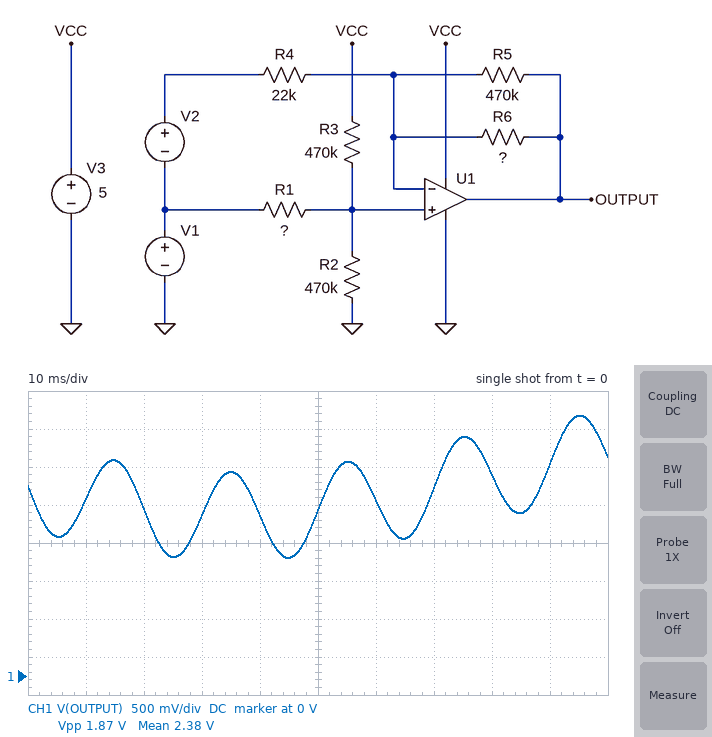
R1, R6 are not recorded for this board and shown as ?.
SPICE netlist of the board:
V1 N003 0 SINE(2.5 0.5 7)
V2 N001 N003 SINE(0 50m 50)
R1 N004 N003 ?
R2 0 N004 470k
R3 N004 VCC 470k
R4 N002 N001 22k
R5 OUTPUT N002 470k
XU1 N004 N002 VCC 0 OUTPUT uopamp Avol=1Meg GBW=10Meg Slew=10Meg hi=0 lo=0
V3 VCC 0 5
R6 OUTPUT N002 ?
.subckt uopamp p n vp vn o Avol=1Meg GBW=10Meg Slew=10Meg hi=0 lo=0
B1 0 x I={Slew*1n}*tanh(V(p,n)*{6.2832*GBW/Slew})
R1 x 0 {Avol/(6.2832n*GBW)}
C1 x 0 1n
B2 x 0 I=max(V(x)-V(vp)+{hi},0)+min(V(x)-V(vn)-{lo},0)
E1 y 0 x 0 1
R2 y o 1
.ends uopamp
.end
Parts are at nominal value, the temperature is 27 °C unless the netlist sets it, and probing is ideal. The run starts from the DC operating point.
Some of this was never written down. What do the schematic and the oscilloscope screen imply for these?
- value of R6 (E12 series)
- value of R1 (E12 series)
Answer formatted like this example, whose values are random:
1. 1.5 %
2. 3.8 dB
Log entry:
1. 560 kΩ
2. 39 kΩ
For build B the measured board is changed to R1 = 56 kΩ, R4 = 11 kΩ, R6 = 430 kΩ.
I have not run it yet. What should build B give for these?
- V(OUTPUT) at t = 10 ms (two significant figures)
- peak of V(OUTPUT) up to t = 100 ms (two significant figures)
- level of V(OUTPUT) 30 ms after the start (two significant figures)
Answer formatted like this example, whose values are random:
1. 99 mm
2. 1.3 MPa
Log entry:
1. 1.8 V
2. 4.9 V
3. 990 mV
